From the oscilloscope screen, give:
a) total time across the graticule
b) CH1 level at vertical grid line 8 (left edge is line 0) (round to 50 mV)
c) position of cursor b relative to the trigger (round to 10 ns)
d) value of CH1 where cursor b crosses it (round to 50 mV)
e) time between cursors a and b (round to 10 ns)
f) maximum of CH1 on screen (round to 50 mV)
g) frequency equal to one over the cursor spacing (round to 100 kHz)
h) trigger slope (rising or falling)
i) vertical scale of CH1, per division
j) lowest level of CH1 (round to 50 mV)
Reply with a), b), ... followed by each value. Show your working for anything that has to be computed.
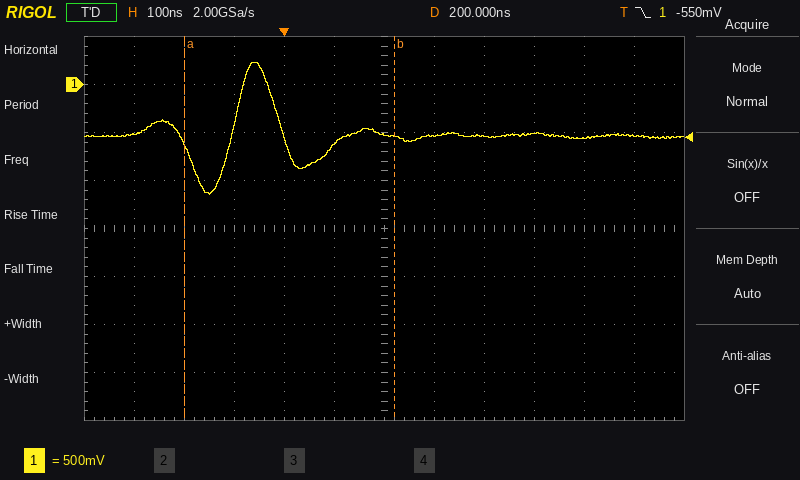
a) 1.2 µs
b) -550 mV
c) +220 ns
d) -550 mV
e) 420 ns
f) 250 mV
g) 1 / 420 ns ≈ 2.4 MHz
h) falling
i) 500 mV
j) -1.15 V
